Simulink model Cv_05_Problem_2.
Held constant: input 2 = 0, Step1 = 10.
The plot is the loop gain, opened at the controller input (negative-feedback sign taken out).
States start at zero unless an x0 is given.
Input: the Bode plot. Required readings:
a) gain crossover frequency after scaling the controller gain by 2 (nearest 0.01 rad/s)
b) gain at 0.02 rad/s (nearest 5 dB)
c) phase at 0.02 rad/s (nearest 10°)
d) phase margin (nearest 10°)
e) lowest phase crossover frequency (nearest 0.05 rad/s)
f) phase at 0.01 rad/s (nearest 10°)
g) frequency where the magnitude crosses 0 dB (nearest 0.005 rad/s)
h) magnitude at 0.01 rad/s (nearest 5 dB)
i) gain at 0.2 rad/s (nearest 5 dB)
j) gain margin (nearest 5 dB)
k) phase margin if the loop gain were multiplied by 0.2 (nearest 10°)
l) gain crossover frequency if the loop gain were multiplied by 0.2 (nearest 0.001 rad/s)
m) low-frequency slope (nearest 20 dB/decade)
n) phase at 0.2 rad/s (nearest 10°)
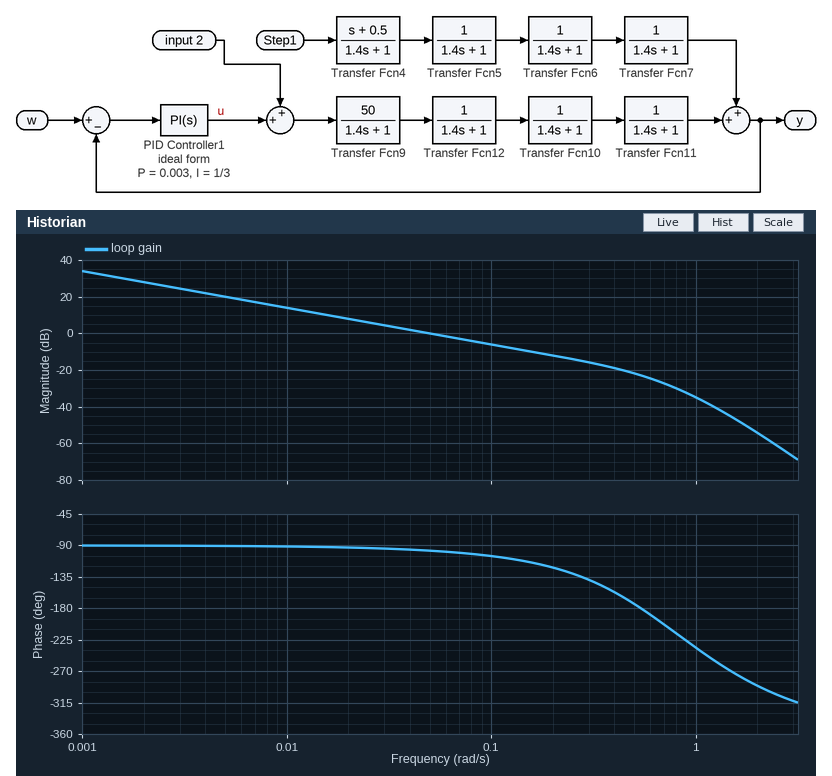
0.10 rad/s
10 dB
-90°
80°
0.55 rad/s
-90°
0.050 rad/s
15 dB
-10 dB
25 dB
90°
0.010 rad/s
-20 dB/decade
-120°
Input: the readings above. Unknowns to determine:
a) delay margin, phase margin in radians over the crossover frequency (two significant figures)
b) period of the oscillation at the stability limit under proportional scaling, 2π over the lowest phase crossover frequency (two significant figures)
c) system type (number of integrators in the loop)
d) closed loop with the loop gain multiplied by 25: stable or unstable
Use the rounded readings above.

28 s
11 s
1
unstable
